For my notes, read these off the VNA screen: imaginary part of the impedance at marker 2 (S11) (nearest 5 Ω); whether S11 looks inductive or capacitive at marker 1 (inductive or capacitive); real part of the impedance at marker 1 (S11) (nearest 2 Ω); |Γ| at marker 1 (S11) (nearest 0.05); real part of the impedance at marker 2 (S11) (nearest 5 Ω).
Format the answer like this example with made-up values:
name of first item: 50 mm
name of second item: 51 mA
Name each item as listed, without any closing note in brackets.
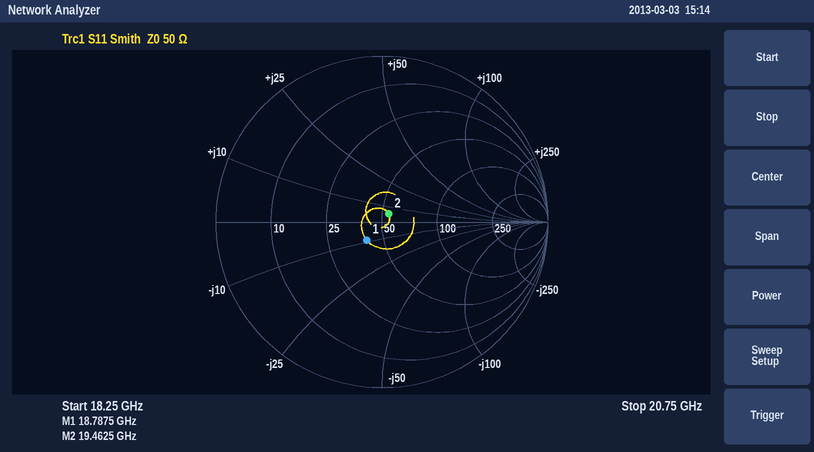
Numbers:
imaginary part of the impedance at marker 2 (S11): +5 Ω
whether S11 looks inductive or capacitive at marker 1: capacitive
real part of the impedance at marker 1 (S11): 40 Ω
|Γ| at marker 1 (S11): 0.15
real part of the impedance at marker 2 (S11): 55 Ω
